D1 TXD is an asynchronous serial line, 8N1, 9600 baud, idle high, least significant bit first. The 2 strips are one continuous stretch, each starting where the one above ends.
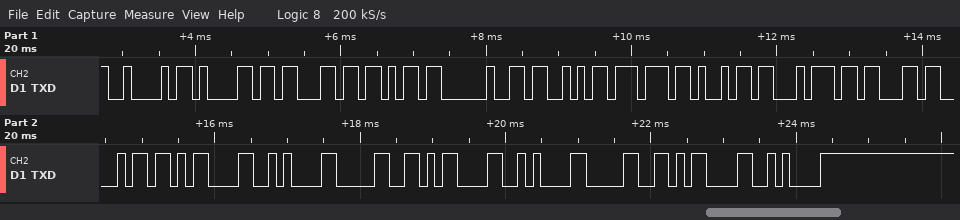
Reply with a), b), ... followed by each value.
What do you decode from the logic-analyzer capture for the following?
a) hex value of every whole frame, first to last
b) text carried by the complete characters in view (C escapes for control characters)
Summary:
a) 42 61 63 6B 20 53 77 69 74 63 68 0D 0A 30 0D 0A 30 0D 0A
b) "Back Switch\r\n0\r\n0\r\n"
